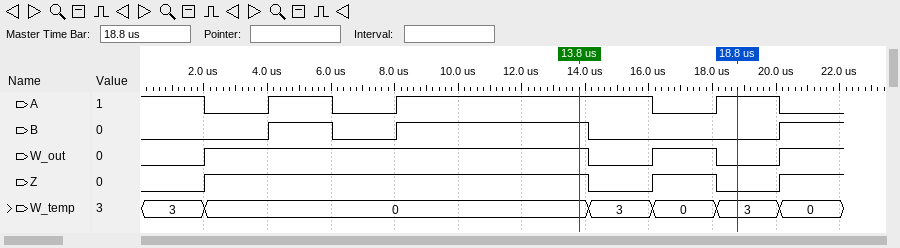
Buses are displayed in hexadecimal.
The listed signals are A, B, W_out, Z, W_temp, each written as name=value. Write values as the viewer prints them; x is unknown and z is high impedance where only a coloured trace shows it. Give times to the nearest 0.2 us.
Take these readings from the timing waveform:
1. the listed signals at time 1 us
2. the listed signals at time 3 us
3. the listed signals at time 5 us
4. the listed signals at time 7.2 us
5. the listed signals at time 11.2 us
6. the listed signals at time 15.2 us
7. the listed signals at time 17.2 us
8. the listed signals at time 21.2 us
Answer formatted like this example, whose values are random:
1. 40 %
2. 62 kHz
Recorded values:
1. A=1, B=0, W_out=0, Z=0, W_temp=3
2. A=0, B=0, W_out=1, Z=1, W_temp=0
3. A=1, B=1, W_out=1, Z=1, W_temp=0
4. A=0, B=0, W_out=1, Z=1, W_temp=0
5. A=1, B=1, W_out=1, Z=1, W_temp=0
6. A=1, B=0, W_out=0, Z=0, W_temp=3
7. A=0, B=0, W_out=1, Z=1, W_temp=0
8. A=0, B=1, W_out=1, Z=1, W_temp=0
